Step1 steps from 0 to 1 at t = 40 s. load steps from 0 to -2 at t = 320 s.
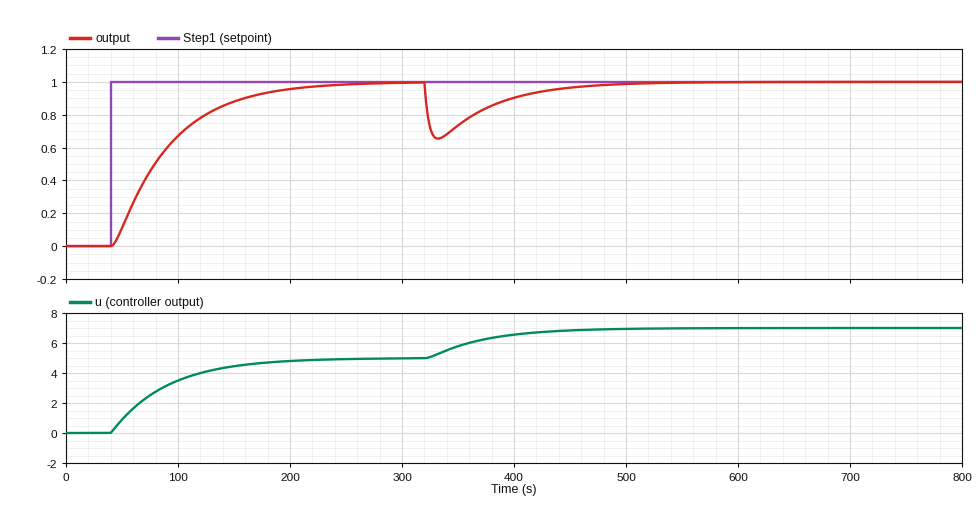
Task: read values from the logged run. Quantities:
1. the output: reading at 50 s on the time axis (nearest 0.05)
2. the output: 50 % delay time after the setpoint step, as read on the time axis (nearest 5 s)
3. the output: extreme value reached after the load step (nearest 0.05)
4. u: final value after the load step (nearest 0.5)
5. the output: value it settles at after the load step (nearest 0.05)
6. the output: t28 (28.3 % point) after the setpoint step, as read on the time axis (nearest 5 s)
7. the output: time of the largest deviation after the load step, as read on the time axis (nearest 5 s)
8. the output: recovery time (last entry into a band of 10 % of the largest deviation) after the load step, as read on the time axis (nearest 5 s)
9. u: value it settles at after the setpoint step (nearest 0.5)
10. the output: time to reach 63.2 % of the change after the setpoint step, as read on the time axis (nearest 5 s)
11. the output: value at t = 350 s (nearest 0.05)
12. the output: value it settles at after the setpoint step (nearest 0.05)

0.10
80 s
0.65
7.0
1.00
60 s
330 s
450 s
5.0
95 s
0.75
1.00
